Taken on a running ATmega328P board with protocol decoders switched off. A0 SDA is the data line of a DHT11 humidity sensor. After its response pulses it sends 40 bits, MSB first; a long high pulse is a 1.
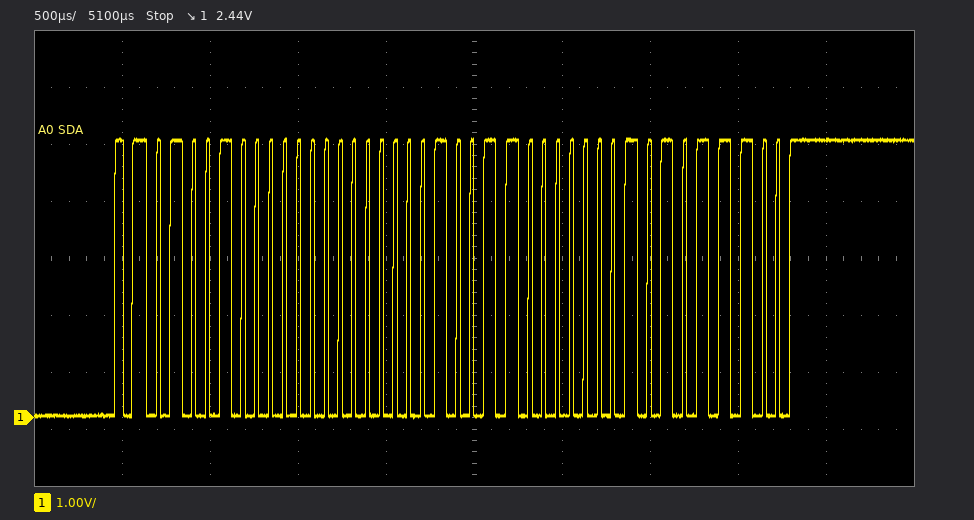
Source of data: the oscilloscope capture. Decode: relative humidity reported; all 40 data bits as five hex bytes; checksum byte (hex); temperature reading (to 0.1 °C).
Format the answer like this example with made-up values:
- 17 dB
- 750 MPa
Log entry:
- 72 %
- 48 00 13 01 5C
- 0x5C
- 19.1 °C
